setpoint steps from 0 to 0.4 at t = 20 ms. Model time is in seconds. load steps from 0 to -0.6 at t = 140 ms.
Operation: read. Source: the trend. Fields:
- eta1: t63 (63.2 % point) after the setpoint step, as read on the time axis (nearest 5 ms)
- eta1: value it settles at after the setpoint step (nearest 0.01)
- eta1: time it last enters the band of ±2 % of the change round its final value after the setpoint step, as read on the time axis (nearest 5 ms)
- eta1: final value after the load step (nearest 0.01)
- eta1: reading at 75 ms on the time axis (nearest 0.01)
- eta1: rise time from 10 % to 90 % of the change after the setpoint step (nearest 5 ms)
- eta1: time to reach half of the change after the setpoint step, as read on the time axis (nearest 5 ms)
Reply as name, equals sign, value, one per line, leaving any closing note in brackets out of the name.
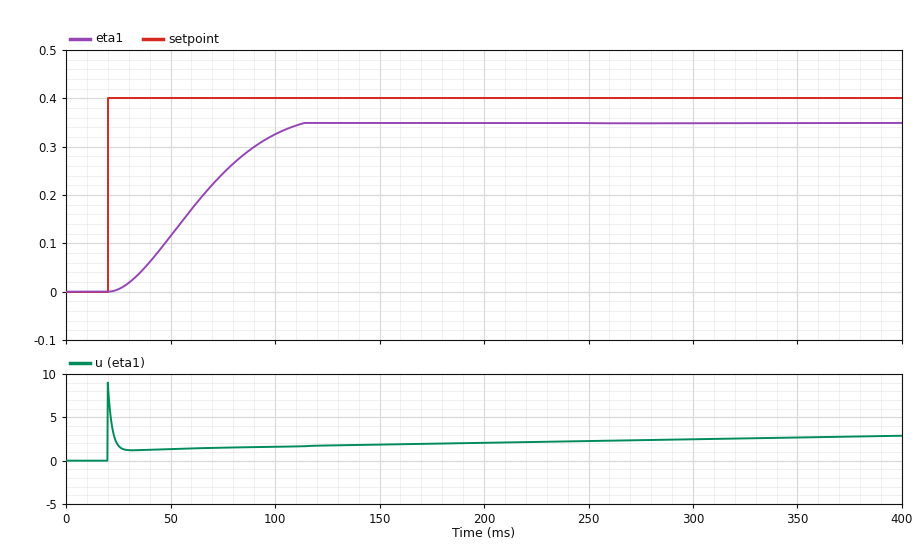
eta1: t63 (63.2 % point) after the setpoint step, as read on the time axis = 70 ms
eta1: value it settles at after the setpoint step = 0.35
eta1: time it last enters the band of ±2 % of the change round its final value after the setpoint step, as read on the time axis = 110 ms
eta1: final value after the load step = 0.35
eta1: reading at 75 ms on the time axis = 0.24
eta1: rise time from 10 % to 90 % of the change after the setpoint step = 60 ms
eta1: time to reach half of the change after the setpoint step, as read on the time axis = 60 ms
